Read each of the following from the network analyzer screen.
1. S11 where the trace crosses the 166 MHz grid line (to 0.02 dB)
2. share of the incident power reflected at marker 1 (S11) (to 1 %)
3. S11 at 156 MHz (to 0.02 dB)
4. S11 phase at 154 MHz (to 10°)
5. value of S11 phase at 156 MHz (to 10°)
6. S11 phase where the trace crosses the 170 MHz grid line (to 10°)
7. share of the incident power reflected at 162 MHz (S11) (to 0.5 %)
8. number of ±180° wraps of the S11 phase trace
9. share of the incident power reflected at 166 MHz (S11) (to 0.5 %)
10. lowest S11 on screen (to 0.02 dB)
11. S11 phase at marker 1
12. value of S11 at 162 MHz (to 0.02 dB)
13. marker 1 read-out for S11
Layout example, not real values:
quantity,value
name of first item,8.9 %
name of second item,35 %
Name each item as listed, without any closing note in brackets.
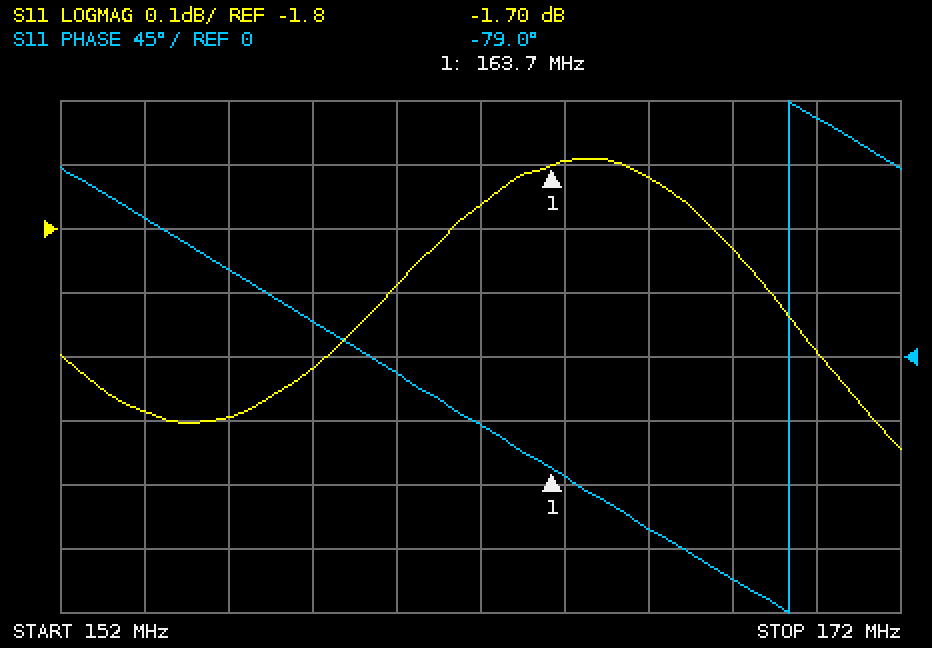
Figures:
quantity,value
S11 where the trace crosses the 166 MHz grid line,-1.72 dB
share of the incident power reflected at marker 1 (S11),68 %
S11 at 156 MHz,-2.10 dB
S11 phase at 154 MHz,100°
value of S11 phase at 156 MHz,60°
S11 phase where the trace crosses the 170 MHz grid line,170°
share of the incident power reflected at 162 MHz (S11),66.5 %
number of ±180° wraps of the S11 phase trace,1
share of the incident power reflected at 166 MHz (S11),67.5 %
lowest S11 on screen,-2.14 dB
S11 phase at marker 1,-79.0°
value of S11 at 162 MHz,-1.76 dB
marker 1 read-out for S11,-1.70 dB
